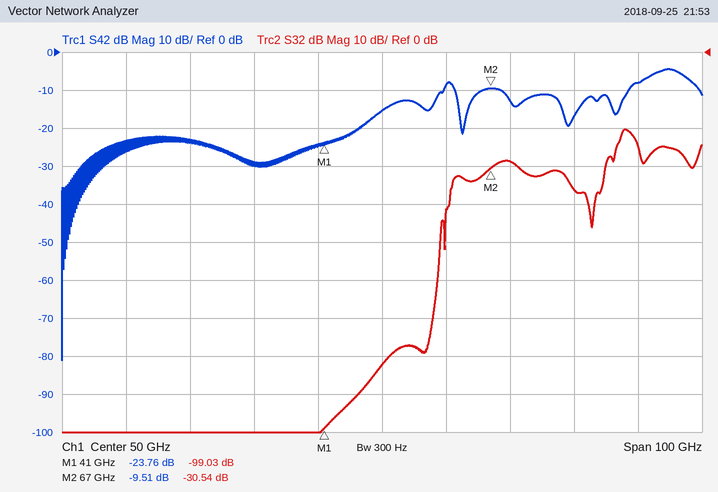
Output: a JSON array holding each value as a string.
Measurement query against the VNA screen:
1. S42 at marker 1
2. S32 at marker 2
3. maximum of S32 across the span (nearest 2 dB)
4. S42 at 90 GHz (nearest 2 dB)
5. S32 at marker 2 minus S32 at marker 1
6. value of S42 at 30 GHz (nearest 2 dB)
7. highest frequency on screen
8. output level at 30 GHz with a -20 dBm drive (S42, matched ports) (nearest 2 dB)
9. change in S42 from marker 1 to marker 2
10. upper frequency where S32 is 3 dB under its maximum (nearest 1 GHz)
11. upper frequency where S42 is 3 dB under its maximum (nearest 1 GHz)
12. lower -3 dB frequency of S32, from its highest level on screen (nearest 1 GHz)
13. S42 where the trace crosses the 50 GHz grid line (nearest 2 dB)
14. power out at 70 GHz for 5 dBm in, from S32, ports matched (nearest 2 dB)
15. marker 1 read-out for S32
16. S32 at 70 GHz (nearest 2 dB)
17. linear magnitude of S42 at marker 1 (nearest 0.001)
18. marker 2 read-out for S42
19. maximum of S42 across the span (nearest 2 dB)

["-23.76 dB", "-30.54 dB", "-20 dB", "-8 dB", "68.49 dB", "-30 dB", "100 GHz", "-50 dBm", "14.25 dB", "90 GHz", "98 GHz", "87 GHz", "-16 dB", "-24 dBm", "-99.03 dB", "-28 dB", "0.065", "-9.51 dB", "-4 dB"]
